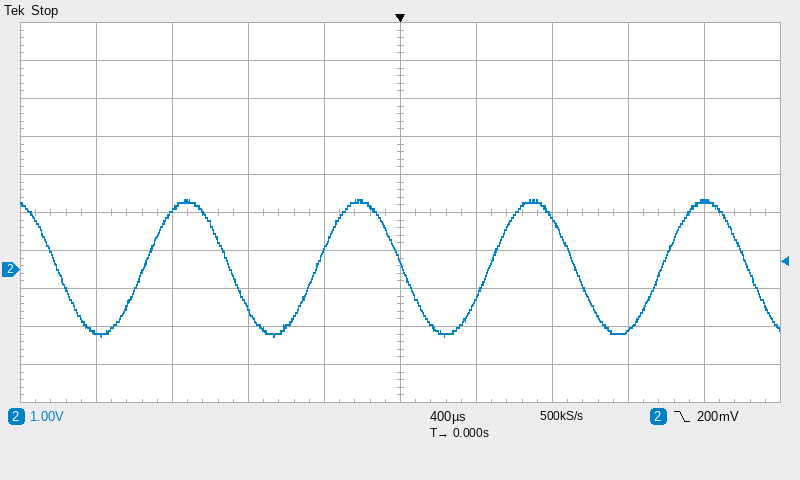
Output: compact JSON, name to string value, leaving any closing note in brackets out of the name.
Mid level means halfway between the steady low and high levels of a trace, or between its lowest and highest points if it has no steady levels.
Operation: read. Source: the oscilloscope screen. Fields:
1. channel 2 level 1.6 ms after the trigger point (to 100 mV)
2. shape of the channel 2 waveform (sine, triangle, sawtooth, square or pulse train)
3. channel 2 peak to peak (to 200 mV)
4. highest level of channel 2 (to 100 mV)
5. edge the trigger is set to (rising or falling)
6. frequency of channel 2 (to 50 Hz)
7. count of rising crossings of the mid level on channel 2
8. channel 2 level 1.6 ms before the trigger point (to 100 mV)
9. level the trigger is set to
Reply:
{"channel 2 level 1.6 ms after the trigger point": "1.8 V", "shape of the channel 2 waveform": "sine", "channel 2 peak to peak": "3.6 V", "highest level of channel 2": "1.8 V", "edge the trigger is set to": "falling", "frequency of channel 2": "1.10 kHz", "count of rising crossings of the mid level on channel 2": "4", "channel 2 level 1.6 ms before the trigger point": "-1.6 V", "level the trigger is set to": "200 mV"}
